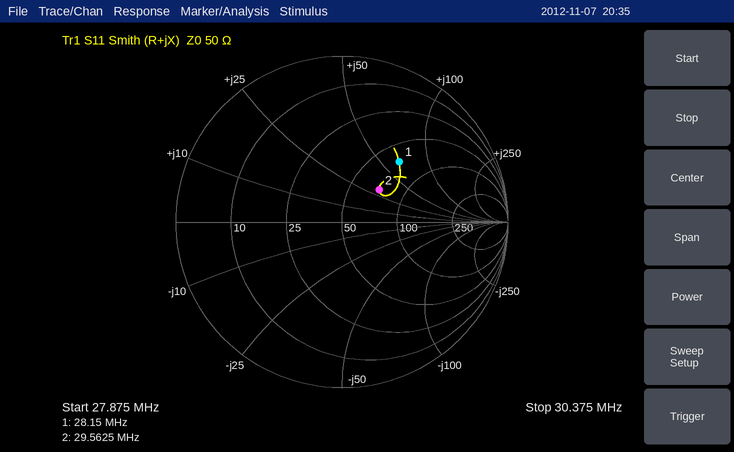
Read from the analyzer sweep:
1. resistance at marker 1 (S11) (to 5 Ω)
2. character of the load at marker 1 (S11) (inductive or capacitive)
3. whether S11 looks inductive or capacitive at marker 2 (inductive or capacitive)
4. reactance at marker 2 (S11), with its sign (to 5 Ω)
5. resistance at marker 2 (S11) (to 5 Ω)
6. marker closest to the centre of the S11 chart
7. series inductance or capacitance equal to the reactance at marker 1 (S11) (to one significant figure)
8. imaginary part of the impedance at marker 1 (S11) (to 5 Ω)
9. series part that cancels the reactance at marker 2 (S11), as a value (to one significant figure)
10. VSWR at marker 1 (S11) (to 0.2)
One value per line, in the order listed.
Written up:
65 Ω
inductive
inductive
+30 Ω
70 Ω
marker 2
400 nH
+65 Ω
200 pF
3.0
